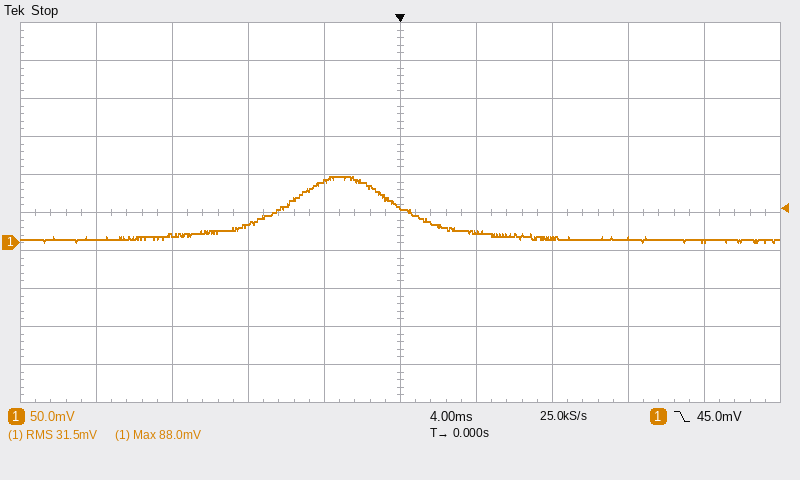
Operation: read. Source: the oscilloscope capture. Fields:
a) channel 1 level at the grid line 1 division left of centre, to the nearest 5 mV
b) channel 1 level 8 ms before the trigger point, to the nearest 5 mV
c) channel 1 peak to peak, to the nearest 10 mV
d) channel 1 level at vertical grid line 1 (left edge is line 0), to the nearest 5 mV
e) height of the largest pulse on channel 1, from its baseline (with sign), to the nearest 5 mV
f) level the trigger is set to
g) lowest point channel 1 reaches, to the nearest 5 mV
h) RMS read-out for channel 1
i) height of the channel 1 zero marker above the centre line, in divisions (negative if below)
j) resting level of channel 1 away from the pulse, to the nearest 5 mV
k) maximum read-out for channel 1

80 mV
25 mV
90 mV
5 mV
+85 mV
45.0 mV
0 mV
31.5 mV
-0.8 div
5 mV
88.0 mV
